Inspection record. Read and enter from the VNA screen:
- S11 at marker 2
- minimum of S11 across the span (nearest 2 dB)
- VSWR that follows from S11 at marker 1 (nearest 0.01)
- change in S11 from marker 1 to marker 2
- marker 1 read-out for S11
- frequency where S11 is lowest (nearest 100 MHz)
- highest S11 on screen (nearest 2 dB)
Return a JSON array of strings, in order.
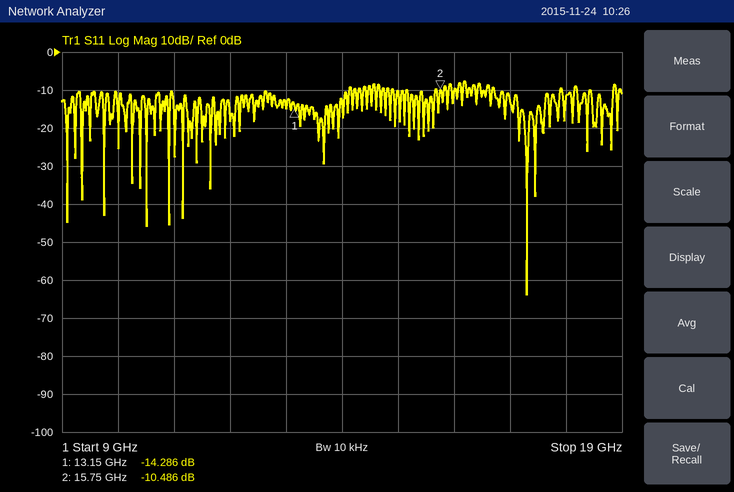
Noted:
["-10.486 dB", "-64 dB", "1.48", "3.800 dB", "-14.286 dB", "17.3 GHz", "-8 dB"]
